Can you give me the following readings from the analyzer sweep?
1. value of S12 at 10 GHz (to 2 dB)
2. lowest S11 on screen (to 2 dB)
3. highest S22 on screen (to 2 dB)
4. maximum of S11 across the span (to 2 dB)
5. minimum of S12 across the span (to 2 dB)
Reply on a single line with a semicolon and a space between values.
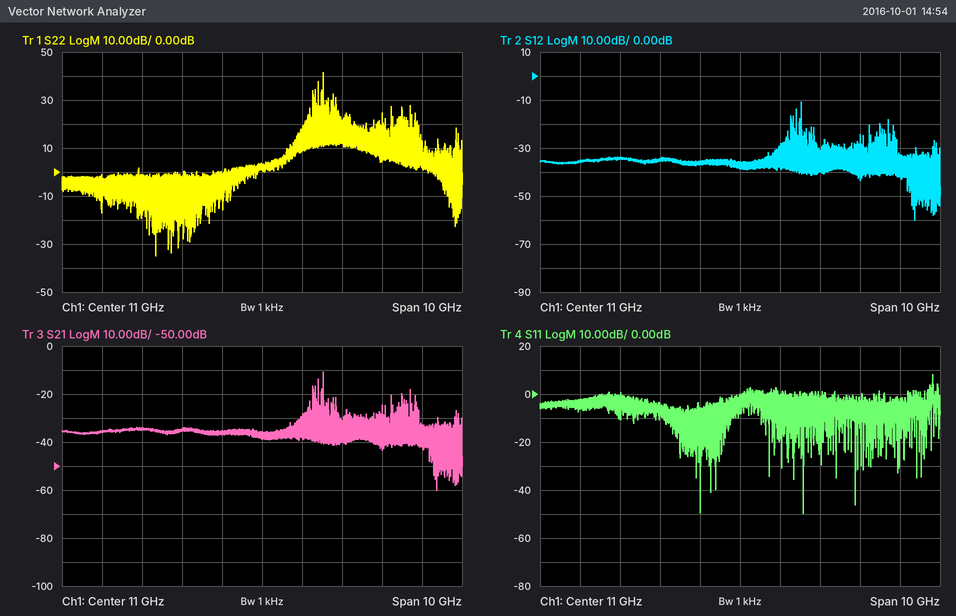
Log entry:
-36 dB; -50 dB; 42 dB; 8 dB; -60 dB
